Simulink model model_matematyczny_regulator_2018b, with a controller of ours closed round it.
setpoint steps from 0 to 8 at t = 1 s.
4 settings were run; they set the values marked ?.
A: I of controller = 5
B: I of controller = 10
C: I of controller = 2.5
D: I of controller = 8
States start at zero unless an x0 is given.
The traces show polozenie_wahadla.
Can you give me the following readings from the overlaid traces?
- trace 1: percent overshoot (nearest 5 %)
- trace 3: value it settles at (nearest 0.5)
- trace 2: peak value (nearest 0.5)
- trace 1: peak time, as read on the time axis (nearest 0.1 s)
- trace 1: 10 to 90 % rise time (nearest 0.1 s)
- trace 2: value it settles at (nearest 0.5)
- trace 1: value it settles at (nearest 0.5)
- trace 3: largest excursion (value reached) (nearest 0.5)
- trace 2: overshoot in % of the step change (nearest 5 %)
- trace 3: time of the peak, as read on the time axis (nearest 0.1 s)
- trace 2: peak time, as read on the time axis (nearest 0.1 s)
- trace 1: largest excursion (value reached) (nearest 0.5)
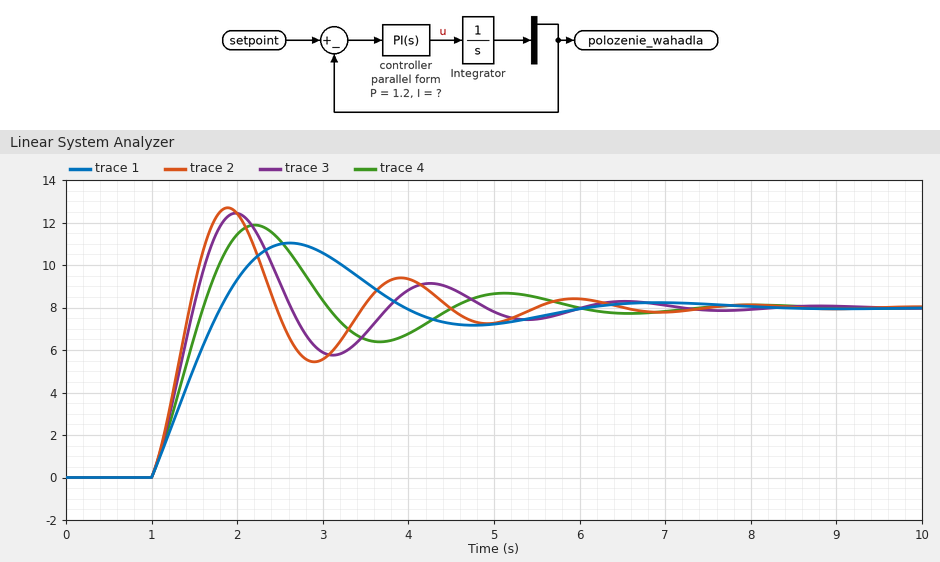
40 %
8.0
12.5
2.6 s
0.6 s
8.0
8.0
12.5
60 %
2.0 s
1.9 s
11.0
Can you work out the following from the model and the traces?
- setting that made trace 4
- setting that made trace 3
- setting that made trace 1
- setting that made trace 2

A
D
C
B
